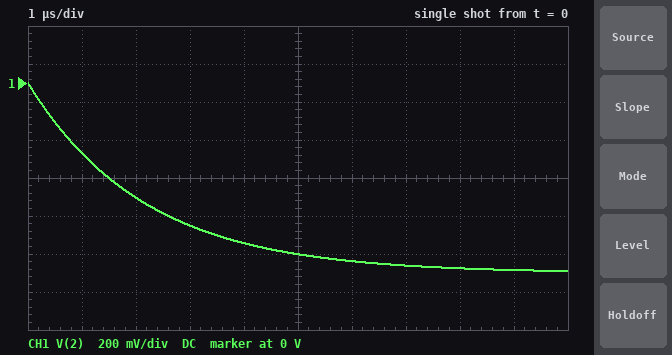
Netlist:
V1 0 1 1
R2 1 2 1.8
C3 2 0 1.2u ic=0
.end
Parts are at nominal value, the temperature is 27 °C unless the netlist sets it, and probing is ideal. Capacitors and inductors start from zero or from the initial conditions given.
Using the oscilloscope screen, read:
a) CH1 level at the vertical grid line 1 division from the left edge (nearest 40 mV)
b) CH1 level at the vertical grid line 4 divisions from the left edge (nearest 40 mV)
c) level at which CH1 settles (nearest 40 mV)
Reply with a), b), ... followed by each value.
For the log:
a) -360 mV
b) -840 mV
c) -1.00 V
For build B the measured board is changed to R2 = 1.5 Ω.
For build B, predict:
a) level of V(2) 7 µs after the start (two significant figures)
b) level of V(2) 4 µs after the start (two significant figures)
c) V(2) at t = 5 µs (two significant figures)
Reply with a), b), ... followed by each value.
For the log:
a) -980 mV
b) -890 mV
c) -940 mV
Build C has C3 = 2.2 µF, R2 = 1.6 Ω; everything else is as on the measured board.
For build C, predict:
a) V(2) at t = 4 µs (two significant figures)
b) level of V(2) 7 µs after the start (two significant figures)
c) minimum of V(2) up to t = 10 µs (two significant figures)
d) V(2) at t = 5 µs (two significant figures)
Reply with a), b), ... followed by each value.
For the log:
a) -680 mV
b) -860 mV
c) -940 mV
d) -760 mV
